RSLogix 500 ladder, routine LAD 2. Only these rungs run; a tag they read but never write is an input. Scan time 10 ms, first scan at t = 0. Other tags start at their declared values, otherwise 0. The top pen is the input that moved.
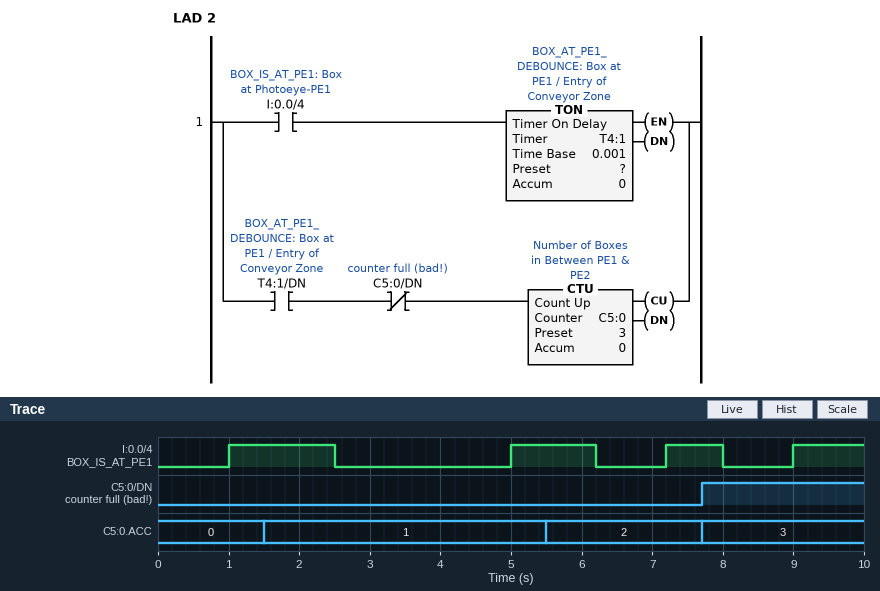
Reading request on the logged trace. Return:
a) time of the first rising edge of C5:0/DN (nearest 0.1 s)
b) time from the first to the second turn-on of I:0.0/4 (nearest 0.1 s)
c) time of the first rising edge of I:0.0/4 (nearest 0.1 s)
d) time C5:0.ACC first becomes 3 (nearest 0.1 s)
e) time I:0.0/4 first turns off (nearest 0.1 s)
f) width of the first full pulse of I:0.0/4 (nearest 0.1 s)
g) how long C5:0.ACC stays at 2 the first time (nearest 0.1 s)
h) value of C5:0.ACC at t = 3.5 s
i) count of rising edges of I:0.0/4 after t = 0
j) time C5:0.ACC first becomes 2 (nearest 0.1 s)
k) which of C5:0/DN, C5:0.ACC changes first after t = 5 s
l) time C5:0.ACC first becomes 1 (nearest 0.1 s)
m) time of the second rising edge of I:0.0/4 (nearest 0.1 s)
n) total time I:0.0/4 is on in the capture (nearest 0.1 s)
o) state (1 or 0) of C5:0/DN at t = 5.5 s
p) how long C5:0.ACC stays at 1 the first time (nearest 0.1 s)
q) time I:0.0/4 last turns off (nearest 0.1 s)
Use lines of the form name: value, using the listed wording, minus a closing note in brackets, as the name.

time of the first rising edge of C5:0/DN: 7.7 s
time from the first to the second turn-on of I:0.0/4: 4.0 s
time of the first rising edge of I:0.0/4: 1.0 s
time C5:0.ACC first becomes 3: 7.7 s
time I:0.0/4 first turns off: 2.5 s
width of the first full pulse of I:0.0/4: 1.5 s
how long C5:0.ACC stays at 2 the first time: 2.2 s
value of C5:0.ACC at t = 3.5 s: 1
count of rising edges of I:0.0/4 after t = 0: 4
time C5:0.ACC first becomes 2: 5.5 s
which of C5:0/DN, C5:0.ACC changes first after t = 5 s: C5:0.ACC
time C5:0.ACC first becomes 1: 1.5 s
time of the second rising edge of I:0.0/4: 5.0 s
total time I:0.0/4 is on in the capture: 4.5 s
state (1 or 0) of C5:0/DN at t = 5.5 s: 0
how long C5:0.ACC stays at 1 the first time: 4.0 s
time I:0.0/4 last turns off: 8.0 s
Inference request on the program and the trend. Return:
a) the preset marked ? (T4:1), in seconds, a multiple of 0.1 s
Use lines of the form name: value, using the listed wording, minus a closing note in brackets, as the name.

the preset marked ? (T4:1), in seconds, a multiple of 0.1 s: 0.5 s
